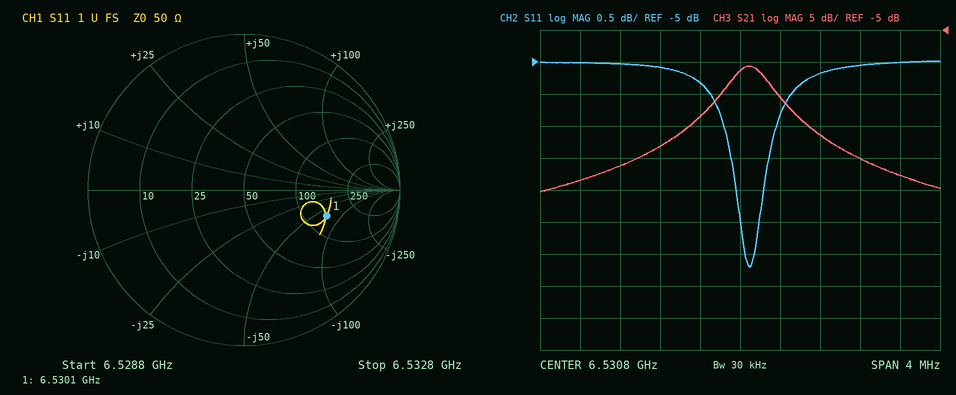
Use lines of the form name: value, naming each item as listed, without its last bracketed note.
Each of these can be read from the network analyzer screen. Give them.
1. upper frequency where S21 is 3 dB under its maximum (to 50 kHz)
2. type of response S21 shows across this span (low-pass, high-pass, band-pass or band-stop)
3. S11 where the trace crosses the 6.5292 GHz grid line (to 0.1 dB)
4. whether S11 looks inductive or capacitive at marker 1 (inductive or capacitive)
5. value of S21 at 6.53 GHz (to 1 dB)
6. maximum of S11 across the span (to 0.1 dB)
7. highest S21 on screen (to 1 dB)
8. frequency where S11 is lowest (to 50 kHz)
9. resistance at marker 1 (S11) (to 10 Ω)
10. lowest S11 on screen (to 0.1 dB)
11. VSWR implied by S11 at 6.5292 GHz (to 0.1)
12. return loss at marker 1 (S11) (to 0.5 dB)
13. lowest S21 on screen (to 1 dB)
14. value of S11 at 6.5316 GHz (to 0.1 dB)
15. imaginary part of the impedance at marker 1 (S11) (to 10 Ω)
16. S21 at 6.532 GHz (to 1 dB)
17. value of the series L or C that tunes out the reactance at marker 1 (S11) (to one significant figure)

upper frequency where S21 is 3 dB under its maximum: 6.53110 GHz
type of response S21 shows across this span: band-pass
S11 where the trace crosses the 6.5292 GHz grid line: -5.0 dB
whether S11 looks inductive or capacitive at marker 1: capacitive
value of S21 at 6.53 GHz: -23 dB
maximum of S11 across the span: -5.0 dB
highest S21 on screen: -11 dB
frequency where S11 is lowest: 6.53090 GHz
resistance at marker 1 (S11): 140 Ω
lowest S11 on screen: -8.2 dB
VSWR implied by S11 at 6.5292 GHz: 3.6
return loss at marker 1 (S11): 5.0 dB
lowest S21 on screen: -30 dB
value of S11 at 6.5316 GHz: -5.2 dB
imaginary part of the impedance at marker 1 (S11): -70 Ω
S21 at 6.532 GHz: -25 dB
value of the series L or C that tunes out the reactance at marker 1 (S11): 2 nH
